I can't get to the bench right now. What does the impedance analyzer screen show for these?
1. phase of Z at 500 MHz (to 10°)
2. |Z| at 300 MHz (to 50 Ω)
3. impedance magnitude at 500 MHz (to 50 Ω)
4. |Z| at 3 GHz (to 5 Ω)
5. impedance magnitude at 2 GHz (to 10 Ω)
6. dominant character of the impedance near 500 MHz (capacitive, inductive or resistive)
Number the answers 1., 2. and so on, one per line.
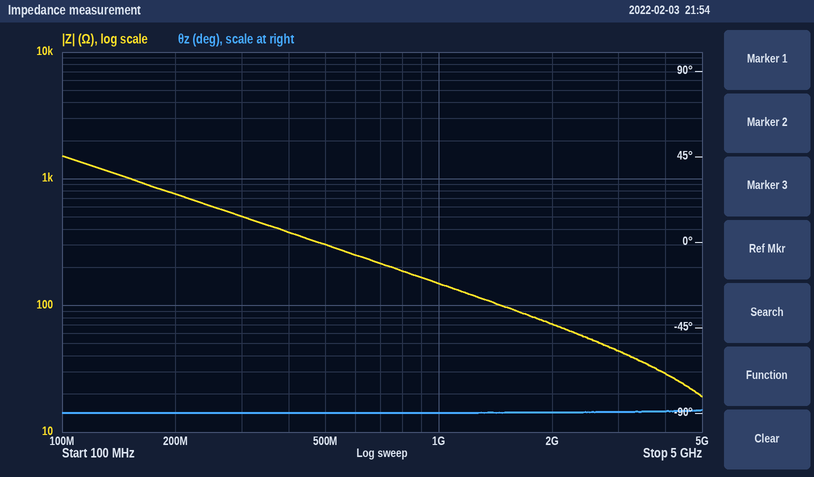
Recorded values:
1. -90°
2. 500 Ω
3. 300 Ω
4. 45 Ω
5. 70 Ω
6. capacitive
